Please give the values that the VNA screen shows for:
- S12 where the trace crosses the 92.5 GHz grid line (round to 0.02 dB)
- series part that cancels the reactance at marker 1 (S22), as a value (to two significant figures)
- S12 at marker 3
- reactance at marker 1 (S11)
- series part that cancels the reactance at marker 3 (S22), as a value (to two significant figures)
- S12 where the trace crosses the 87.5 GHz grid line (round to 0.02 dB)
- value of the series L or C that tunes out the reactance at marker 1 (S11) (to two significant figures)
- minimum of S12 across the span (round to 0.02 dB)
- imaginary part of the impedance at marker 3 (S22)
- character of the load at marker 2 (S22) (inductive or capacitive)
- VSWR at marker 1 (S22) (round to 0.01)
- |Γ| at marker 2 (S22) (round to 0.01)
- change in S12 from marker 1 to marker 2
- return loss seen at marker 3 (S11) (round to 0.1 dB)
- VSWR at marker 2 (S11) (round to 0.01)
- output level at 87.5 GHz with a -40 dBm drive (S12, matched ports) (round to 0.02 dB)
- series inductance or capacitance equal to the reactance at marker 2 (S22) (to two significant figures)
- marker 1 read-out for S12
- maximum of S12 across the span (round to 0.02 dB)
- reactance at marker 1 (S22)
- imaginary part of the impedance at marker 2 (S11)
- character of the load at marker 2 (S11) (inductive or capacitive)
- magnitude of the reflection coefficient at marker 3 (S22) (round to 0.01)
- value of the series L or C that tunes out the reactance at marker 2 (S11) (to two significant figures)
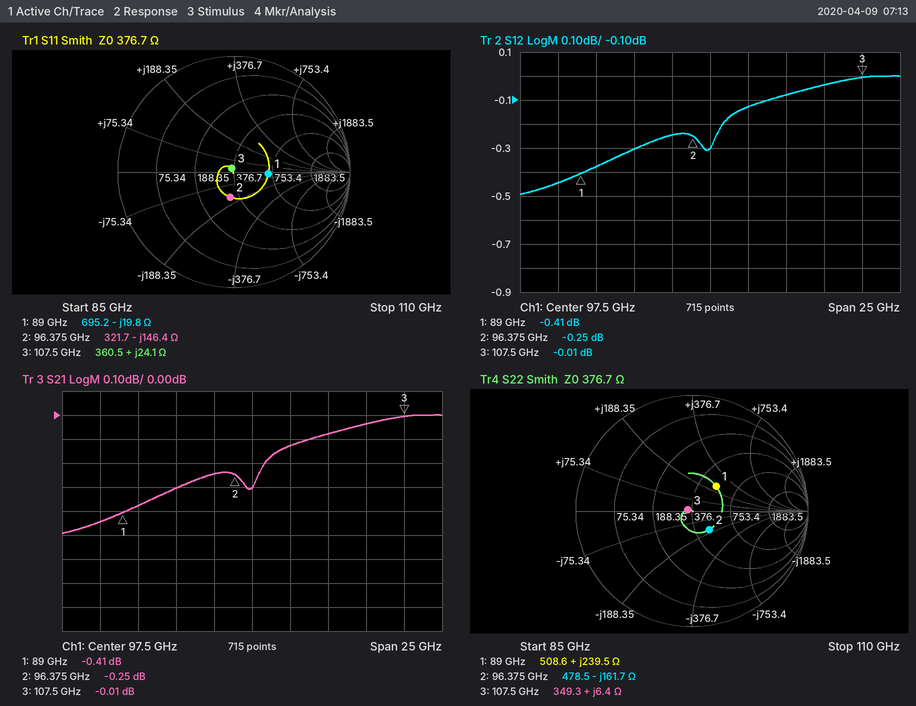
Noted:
-0.30 dB
7.5 fF
-0.01 dB
-19.8 Ω
230 fF
-0.44 dB
35 pH
-0.50 dB
+6.4 Ω
capacitive
1.85
0.22
0.16 dB
28.1 dB
1.56
-40.44 dBm
10 fF
-0.41 dB
0.00 dB
+239.5 Ω
-146.4 Ω
capacitive
0.04
240 pH
